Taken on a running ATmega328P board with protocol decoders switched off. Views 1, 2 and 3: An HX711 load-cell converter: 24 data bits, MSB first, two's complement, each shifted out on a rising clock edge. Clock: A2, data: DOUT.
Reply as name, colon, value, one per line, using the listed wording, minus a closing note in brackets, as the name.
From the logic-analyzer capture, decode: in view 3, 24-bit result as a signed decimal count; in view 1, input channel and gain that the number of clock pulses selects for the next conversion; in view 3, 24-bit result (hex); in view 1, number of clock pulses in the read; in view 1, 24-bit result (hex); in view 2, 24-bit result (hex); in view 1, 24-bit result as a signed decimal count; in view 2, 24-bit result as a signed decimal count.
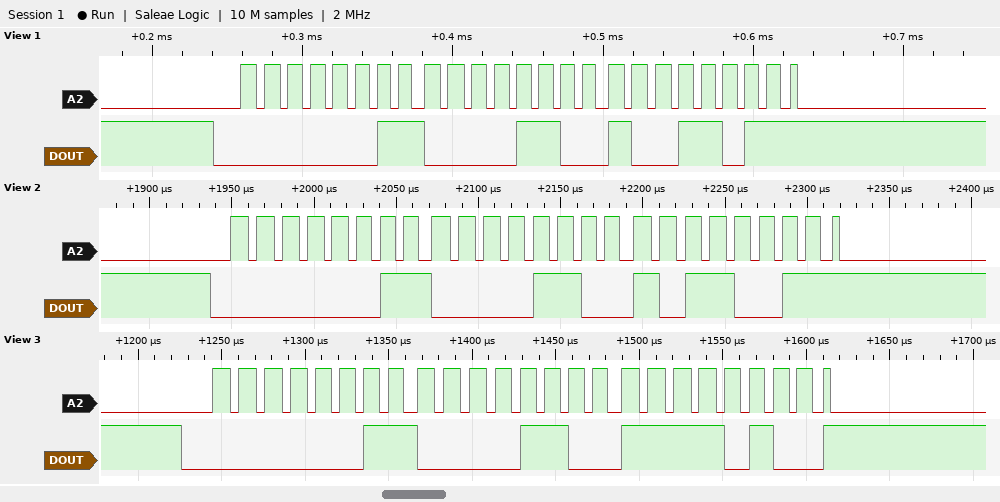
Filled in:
in view 3, 24-bit result as a signed decimal count: 199924
in view 1, input channel and gain that the number of clock pulses selects for the next conversion: channel A, gain 128
in view 3, 24-bit result: 0x030CF4
in view 1, number of clock pulses in the read: 25
in view 1, 24-bit result: 0x030C9B
in view 2, 24-bit result: 0x030CB3
in view 1, 24-bit result as a signed decimal count: 199835
in view 2, 24-bit result as a signed decimal count: 199859
